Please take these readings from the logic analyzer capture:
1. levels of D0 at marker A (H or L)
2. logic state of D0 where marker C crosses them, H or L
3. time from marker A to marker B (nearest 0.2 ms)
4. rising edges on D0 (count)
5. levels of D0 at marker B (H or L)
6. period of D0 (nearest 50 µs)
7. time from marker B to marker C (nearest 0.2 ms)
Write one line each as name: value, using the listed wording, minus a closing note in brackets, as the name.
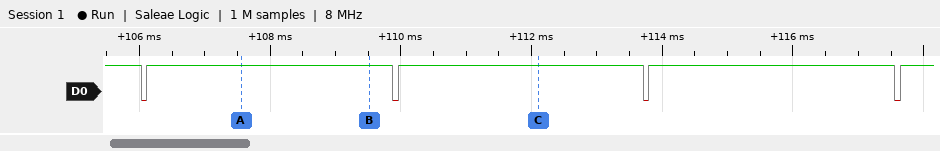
levels of D0 at marker A: D0=H
logic state of D0 where marker C crosses them, H or L: D0=H
time from marker A to marker B: 2 ms
rising edges on D0: 4
levels of D0 at marker B: D0=H
period of D0: 3850 µs
time from marker B to marker C: 2.6 ms
